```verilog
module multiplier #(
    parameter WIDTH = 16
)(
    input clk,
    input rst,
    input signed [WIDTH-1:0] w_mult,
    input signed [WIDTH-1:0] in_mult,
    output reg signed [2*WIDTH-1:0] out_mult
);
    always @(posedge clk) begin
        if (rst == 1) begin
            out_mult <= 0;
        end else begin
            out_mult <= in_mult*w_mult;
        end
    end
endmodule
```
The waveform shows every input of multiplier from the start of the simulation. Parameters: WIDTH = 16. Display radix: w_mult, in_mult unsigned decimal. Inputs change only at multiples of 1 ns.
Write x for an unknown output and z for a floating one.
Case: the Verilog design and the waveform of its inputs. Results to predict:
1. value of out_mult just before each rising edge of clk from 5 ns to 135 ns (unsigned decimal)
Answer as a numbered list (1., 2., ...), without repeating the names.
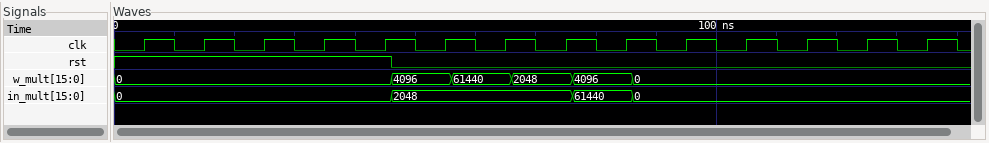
1. x, 0, 0, 0, 0, 0, 8388608, 4286578688, 4194304, 4278190080, 0, 0, 0, 0
